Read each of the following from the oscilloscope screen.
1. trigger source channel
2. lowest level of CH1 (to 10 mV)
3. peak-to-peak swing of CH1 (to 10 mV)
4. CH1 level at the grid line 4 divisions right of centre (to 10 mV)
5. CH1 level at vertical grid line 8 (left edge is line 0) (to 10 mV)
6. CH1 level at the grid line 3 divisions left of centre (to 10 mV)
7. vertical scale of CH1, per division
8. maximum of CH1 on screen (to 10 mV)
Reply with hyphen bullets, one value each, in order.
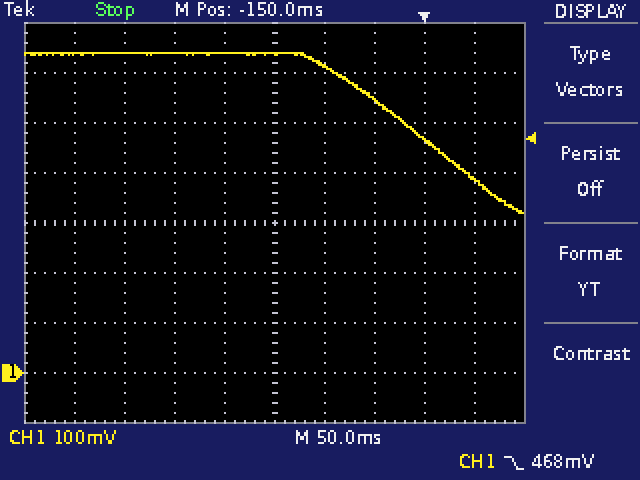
- CH1
- 320 mV
- 320 mV
- 390 mV
- 470 mV
- 640 mV
- 100 mV
- 640 mV
